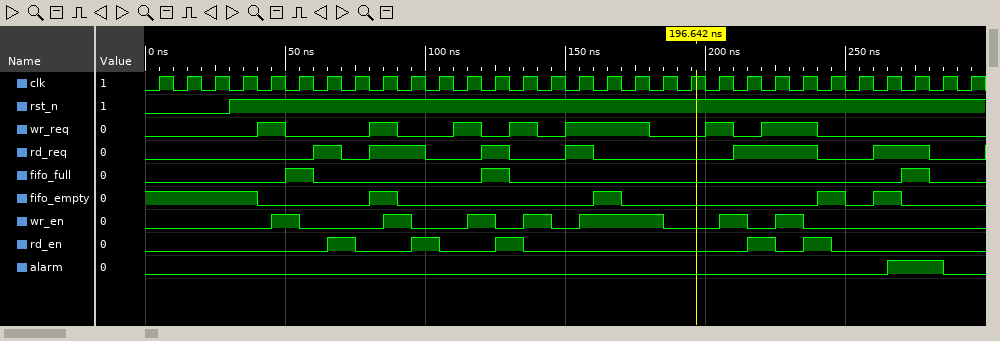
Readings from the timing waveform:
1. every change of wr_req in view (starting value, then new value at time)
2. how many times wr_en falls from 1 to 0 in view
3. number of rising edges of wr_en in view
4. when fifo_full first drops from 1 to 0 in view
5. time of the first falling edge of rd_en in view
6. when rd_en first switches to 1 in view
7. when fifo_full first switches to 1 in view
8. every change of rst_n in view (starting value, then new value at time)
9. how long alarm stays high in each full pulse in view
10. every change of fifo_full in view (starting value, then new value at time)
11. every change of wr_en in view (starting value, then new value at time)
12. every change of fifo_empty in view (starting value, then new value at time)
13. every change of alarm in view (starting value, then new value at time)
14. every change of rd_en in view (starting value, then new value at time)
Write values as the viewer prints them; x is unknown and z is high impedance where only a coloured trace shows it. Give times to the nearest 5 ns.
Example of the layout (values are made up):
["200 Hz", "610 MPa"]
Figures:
["0, 1 at 40 ns, 0 at 50 ns, 1 at 80 ns, 0 at 90 ns, 1 at 110 ns, 0 at 120 ns, 1 at 130 ns, 0 at 140 ns, 1 at 150 ns, 0 at 180 ns, 1 at 200 ns, 0 at 210 ns, 1 at 220 ns, 0 at 240 ns", "7", "7", "60 ns", "75 ns", "65 ns", "50 ns", "0, 1 at 30 ns", "20 ns", "0, 1 at 50 ns, 0 at 60 ns, 1 at 120 ns, 0 at 130 ns, 1 at 270 ns, 0 at 280 ns", "0, 1 at 45 ns, 0 at 55 ns, 1 at 85 ns, 0 at 95 ns, 1 at 115 ns, 0 at 125 ns, 1 at 135 ns, 0 at 145 ns, 1 at 155 ns, 0 at 185 ns, 1 at 205 ns, 0 at 215 ns, 1 at 225 ns, 0 at 235 ns", "1, 0 at 40 ns, 1 at 80 ns, 0 at 90 ns, 1 at 160 ns, 0 at 170 ns, 1 at 240 ns, 0 at 250 ns, 1 at 260 ns, 0 at 270 ns", "0, 1 at 265 ns, 0 at 285 ns", "0, 1 at 65 ns, 0 at 75 ns, 1 at 95 ns, 0 at 105 ns, 1 at 125 ns, 0 at 135 ns, 1 at 215 ns, 0 at 225 ns, 1 at 235 ns, 0 at 245 ns"]
